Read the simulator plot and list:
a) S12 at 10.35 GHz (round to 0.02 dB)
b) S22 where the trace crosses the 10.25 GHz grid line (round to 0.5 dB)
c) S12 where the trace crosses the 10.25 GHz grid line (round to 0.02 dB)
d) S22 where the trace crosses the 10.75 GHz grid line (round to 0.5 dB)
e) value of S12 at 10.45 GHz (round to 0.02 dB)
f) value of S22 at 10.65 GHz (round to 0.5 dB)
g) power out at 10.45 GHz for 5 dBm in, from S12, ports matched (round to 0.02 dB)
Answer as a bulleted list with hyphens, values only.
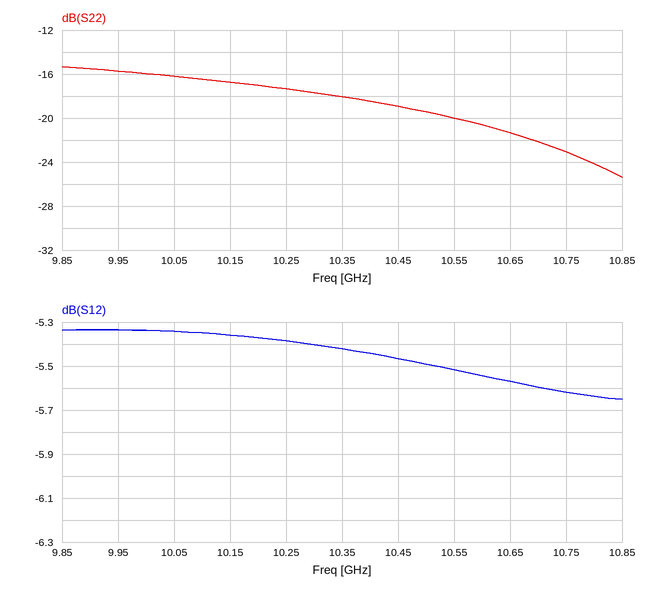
- -5.42 dB
- -17.5 dB
- -5.38 dB
- -23.0 dB
- -5.46 dB
- -21.5 dB
- -0.46 dBm
